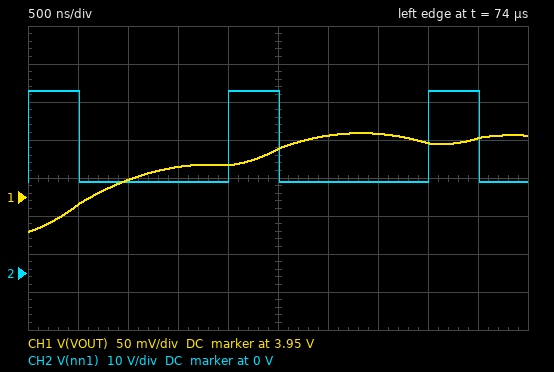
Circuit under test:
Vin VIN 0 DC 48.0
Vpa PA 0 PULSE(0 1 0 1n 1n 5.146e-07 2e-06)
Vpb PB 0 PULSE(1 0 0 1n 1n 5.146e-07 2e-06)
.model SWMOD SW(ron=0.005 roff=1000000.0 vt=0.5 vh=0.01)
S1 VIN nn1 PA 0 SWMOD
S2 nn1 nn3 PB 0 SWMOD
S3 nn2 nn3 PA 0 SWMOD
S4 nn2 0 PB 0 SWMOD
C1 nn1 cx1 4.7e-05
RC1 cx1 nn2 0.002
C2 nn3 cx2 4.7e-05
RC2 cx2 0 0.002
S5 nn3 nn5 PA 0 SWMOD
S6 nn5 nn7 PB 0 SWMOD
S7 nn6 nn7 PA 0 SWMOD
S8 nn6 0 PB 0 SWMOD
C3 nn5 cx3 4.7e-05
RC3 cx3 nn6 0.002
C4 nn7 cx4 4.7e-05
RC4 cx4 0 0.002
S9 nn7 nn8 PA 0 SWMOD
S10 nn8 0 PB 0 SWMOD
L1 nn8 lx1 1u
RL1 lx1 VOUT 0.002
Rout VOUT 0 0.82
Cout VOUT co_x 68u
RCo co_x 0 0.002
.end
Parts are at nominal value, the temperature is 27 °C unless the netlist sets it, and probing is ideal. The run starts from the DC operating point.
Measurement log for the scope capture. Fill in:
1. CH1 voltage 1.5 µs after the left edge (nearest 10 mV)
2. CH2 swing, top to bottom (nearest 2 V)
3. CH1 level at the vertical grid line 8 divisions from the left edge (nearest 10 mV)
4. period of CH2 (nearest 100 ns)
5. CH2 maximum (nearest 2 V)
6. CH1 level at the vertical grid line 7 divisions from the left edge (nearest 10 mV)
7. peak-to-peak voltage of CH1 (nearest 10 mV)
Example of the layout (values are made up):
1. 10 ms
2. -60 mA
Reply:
1. 3.99 V
2. 24 V
3. 4.02 V
4. 2.0 µs
5. 48 V
6. 4.03 V
7. 130 mV
